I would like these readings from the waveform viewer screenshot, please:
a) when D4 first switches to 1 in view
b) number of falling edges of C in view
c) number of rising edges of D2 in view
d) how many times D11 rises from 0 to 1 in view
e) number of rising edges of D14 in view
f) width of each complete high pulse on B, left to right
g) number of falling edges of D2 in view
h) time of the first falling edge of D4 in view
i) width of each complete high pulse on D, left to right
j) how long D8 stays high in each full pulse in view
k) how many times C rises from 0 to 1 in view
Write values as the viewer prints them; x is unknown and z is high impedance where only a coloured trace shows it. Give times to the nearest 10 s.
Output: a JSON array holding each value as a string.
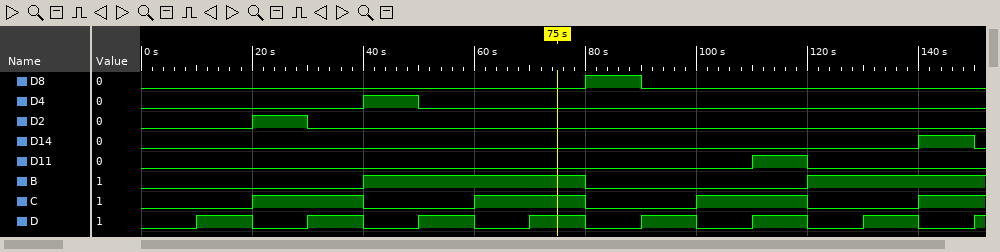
["40 s", "3", "1", "1", "1", "40 s", "1", "50 s", "10 s, 10 s, 10 s, 10 s, 10 s, 10 s, 10 s", "10 s", "4"]
